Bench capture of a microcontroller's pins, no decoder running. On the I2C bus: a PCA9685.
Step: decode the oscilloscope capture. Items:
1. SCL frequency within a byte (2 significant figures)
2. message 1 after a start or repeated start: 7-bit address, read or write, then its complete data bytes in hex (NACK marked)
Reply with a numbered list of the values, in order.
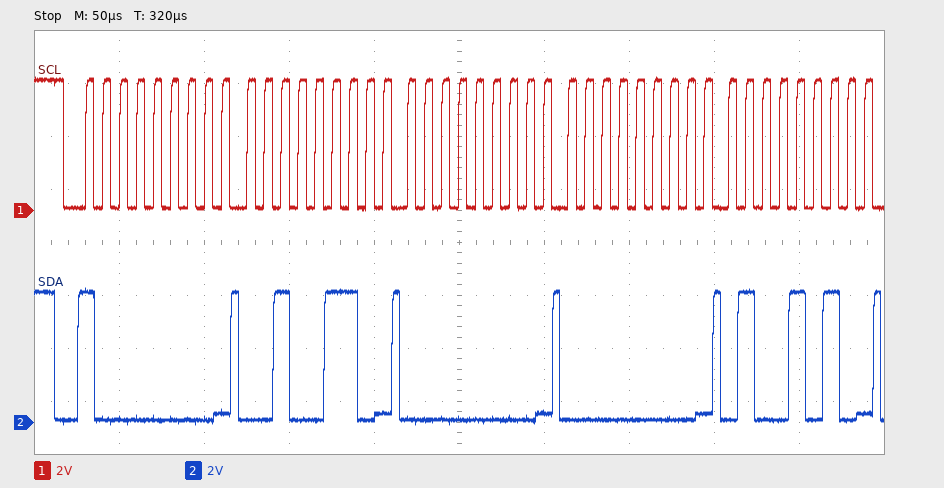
1. 100 kHz
2. 0x40 write: 26 00 00 4A
